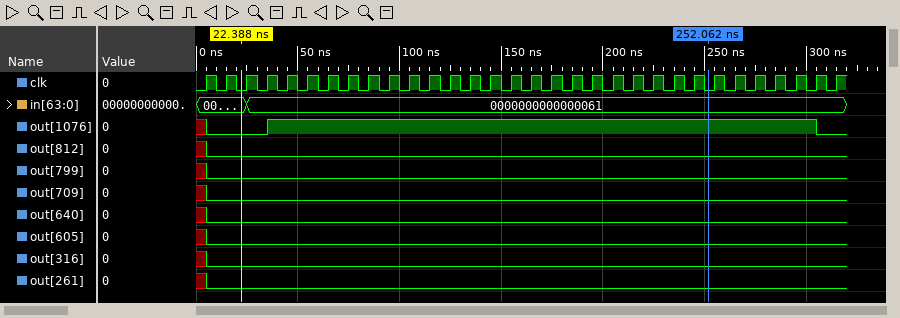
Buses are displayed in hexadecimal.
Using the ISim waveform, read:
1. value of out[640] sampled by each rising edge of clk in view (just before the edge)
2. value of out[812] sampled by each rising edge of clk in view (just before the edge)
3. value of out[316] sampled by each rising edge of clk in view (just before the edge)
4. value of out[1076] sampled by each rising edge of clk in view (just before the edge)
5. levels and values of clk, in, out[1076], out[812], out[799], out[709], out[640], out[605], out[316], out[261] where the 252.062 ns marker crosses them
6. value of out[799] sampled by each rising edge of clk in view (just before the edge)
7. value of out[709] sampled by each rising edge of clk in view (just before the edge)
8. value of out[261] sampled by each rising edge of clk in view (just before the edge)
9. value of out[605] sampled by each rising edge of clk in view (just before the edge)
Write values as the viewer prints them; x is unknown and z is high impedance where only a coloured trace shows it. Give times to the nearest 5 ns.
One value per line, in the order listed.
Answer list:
x 0 0 0 0 0 0 0 0 0 0 0 0 0 0 0 0 0 0 0 0 0 0 0 0 0 0 0 0 0 0 0
x 0 0 0 0 0 0 0 0 0 0 0 0 0 0 0 0 0 0 0 0 0 0 0 0 0 0 0 0 0 0 0
x 0 0 0 0 0 0 0 0 0 0 0 0 0 0 0 0 0 0 0 0 0 0 0 0 0 0 0 0 0 0 0
x 0 0 0 1 1 1 1 1 1 1 1 1 1 1 1 1 1 1 1 1 1 1 1 1 1 1 1 1 1 1 0
clk=0, in=0000000000000061, out[1076]=1, out[812]=0, out[799]=0, out[709]=0, out[640]=0, out[605]=0, out[316]=0, out[261]=0
x 0 0 0 0 0 0 0 0 0 0 0 0 0 0 0 0 0 0 0 0 0 0 0 0 0 0 0 0 0 0 0
x 0 0 0 0 0 0 0 0 0 0 0 0 0 0 0 0 0 0 0 0 0 0 0 0 0 0 0 0 0 0 0
x 0 0 0 0 0 0 0 0 0 0 0 0 0 0 0 0 0 0 0 0 0 0 0 0 0 0 0 0 0 0 0
x 0 0 0 0 0 0 0 0 0 0 0 0 0 0 0 0 0 0 0 0 0 0 0 0 0 0 0 0 0 0 0
